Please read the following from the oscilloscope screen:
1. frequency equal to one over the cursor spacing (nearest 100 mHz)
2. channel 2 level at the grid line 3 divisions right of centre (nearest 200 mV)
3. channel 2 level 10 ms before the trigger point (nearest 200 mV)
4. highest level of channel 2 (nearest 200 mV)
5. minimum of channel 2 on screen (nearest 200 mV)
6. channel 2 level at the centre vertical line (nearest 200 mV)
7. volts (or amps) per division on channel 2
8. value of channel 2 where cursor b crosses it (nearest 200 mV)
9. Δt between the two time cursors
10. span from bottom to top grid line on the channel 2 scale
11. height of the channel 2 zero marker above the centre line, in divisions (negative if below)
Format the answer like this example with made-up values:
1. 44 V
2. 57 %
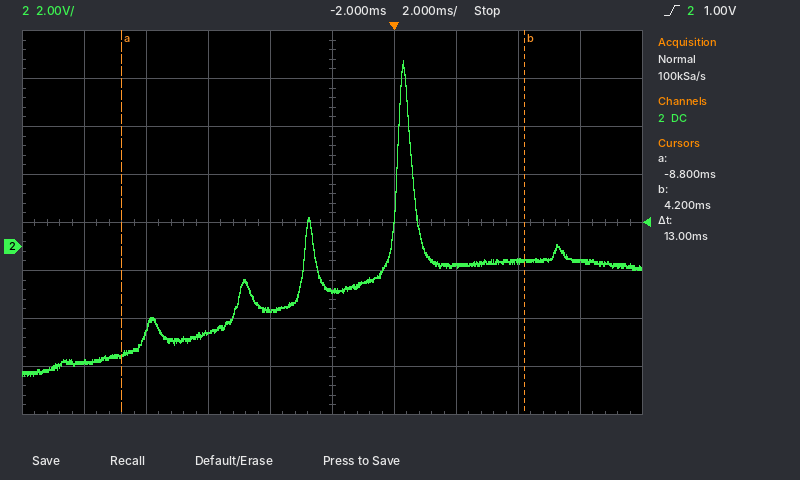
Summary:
1. 76.9 Hz
2. -600 mV
3. -4.8 V
4. 7.8 V
5. -5.4 V
6. -1.8 V
7. 2 V
8. -600 mV
9. 13 ms
10. 16 V
11. -0.5 div
